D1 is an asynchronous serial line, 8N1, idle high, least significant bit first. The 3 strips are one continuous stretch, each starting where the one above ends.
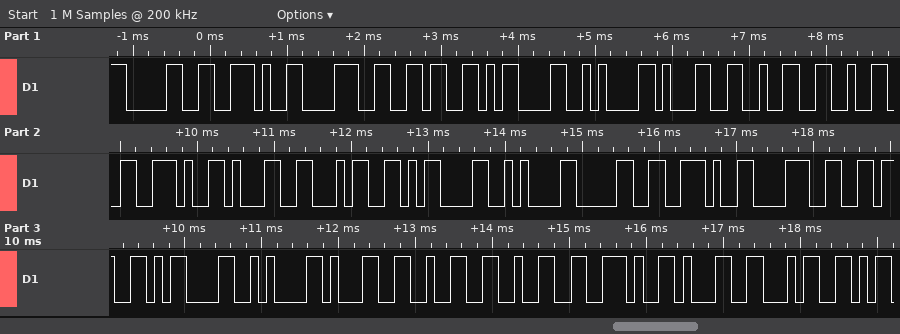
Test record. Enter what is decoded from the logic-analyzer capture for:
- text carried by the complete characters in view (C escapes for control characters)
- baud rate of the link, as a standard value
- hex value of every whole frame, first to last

"0.86\r\n122.14\r\n0.86\r\n122.14"
9600 baud
30 2E 38 36 0D 0A 31 32 32 2E 31 34 0D 0A 30 2E 38 36 0D 0A 31 32 32 2E 31 34
